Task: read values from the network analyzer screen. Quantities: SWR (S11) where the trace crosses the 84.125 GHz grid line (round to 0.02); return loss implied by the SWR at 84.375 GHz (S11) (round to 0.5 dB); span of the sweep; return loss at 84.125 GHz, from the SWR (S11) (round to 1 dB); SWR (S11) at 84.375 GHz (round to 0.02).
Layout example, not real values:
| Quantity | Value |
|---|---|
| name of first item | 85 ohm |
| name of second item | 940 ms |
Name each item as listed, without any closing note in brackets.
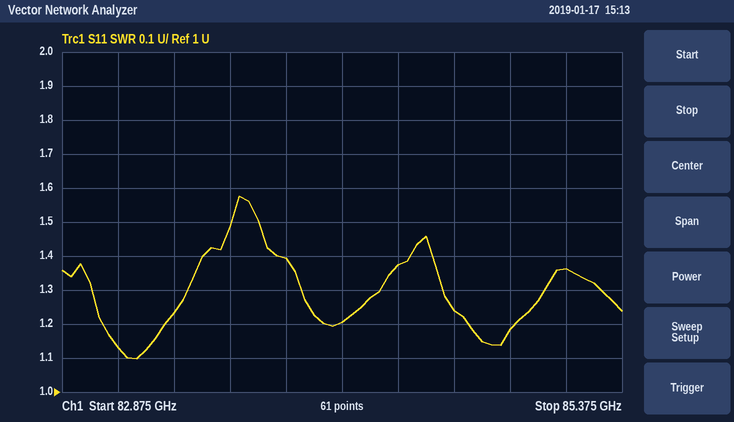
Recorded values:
| Quantity | Value |
|---|---|
| SWR (S11) where the trace crosses the 84.125 GHz grid line | 1.20 |
| return loss implied by the SWR at 84.375 GHz (S11) | 16.0 dB |
| span of the sweep | 2.5 GHz |
| return loss at 84.125 GHz, from the SWR (S11) | 21 dB |
| SWR (S11) at 84.375 GHz | 1.38 |
